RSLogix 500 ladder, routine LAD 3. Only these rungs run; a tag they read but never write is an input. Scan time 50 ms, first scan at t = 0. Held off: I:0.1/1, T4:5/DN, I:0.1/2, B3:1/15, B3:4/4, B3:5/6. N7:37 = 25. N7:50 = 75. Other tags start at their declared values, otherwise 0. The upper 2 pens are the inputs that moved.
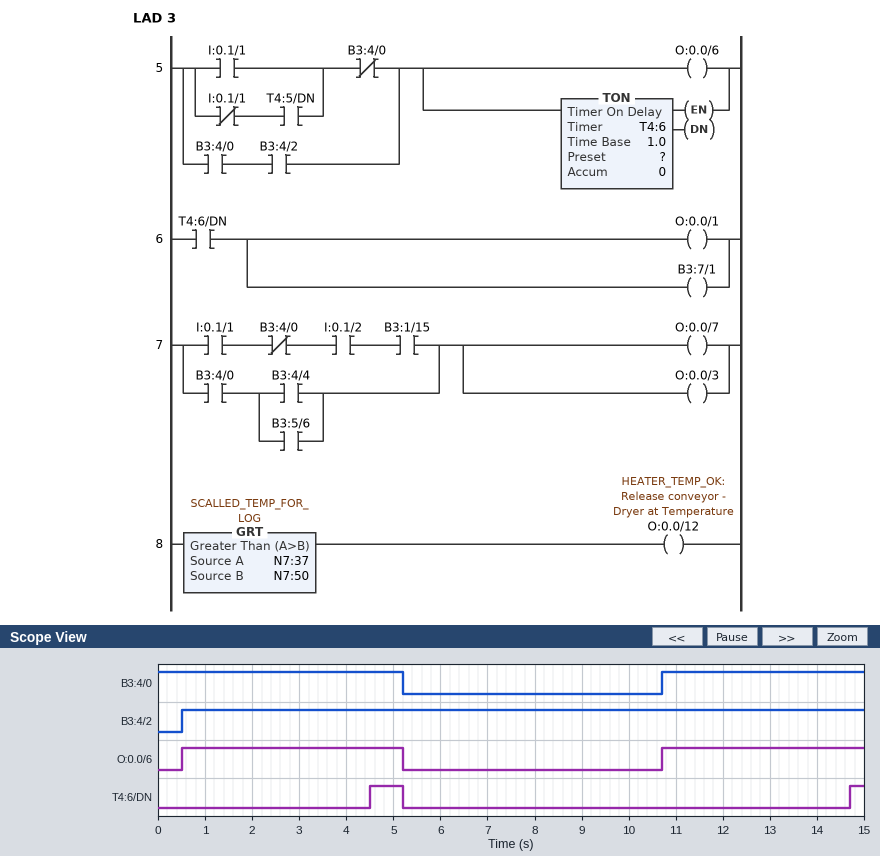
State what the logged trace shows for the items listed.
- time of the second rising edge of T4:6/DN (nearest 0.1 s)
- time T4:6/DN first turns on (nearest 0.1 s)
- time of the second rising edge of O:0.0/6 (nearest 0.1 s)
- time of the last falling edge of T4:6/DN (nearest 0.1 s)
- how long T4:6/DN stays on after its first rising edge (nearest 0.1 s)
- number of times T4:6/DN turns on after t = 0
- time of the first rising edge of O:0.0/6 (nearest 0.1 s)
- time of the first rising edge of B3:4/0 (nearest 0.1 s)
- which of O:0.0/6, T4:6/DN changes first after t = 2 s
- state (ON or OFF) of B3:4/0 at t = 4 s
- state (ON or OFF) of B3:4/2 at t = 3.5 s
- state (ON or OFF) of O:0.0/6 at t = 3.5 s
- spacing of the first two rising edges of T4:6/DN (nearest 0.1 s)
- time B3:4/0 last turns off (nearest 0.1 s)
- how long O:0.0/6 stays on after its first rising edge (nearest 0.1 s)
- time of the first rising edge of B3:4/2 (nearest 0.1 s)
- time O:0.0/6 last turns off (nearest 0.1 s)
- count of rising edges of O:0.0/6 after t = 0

14.7 s
4.5 s
10.7 s
5.2 s
0.7 s
2
0.5 s
10.7 s
T4:6/DN
ON
ON
ON
10.2 s
5.2 s
4.7 s
0.5 s
5.2 s
2
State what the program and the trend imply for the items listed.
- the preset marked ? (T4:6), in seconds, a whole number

4 s
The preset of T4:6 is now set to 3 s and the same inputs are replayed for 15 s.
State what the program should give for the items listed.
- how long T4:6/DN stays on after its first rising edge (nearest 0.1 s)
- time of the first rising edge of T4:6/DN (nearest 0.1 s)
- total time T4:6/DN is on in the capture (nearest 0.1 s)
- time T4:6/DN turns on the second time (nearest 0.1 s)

1.7 s
3.5 s
3.0 s
13.7 s
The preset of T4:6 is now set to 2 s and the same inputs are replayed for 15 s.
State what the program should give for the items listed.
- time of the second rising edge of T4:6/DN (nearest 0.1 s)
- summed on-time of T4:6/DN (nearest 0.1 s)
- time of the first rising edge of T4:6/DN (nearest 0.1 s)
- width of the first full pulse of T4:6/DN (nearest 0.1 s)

12.7 s
5.0 s
2.5 s
2.7 s
